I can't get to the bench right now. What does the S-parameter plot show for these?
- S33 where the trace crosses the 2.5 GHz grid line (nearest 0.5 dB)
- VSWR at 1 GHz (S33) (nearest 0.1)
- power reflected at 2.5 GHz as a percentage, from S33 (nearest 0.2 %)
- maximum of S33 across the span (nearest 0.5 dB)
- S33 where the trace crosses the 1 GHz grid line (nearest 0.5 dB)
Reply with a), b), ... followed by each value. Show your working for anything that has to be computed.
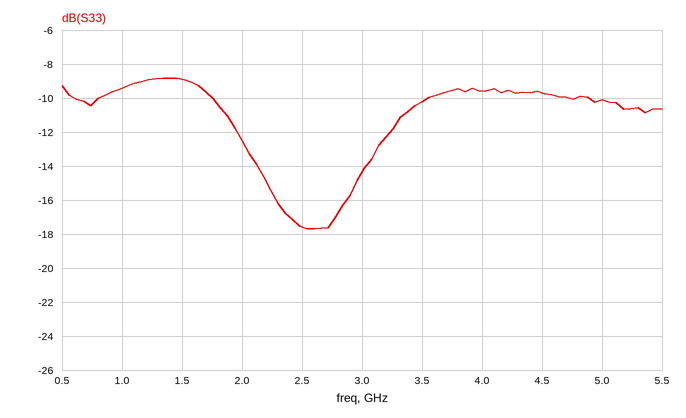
a) -17.5 dB
b) |Γ| = 10^(-9.5/20) = 0.3350; VSWR = (1 + 0.3350)/(1 − 0.3350) ≈ 2.0
c) 10^(-17.5/10) ≈ 1.8 %
d) -9.0 dB
e) -9.5 dB
